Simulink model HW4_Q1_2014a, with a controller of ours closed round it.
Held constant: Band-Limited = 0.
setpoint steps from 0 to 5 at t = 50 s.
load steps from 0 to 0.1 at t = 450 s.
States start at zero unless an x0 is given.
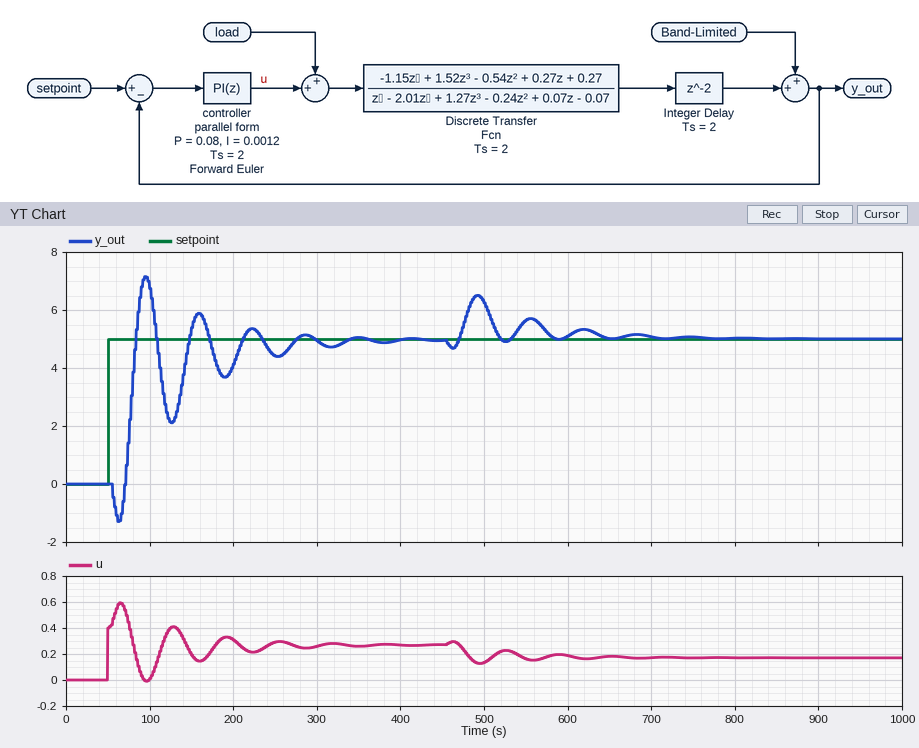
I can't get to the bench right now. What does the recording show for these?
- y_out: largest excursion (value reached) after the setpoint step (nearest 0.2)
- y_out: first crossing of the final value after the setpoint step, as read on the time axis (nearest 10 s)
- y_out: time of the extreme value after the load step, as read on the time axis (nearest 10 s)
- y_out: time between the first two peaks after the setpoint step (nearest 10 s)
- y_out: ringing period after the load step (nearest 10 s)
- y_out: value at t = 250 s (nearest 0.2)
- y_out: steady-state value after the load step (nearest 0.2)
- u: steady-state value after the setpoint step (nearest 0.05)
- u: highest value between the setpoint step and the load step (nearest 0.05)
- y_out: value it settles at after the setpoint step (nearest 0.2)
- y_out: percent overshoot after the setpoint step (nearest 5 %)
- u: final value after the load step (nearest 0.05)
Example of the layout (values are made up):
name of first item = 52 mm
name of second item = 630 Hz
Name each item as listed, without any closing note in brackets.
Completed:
y_out: largest excursion (value reached) after the setpoint step = 7.2
y_out: first crossing of the final value after the setpoint step, as read on the time axis = 80 s
y_out: time of the extreme value after the load step, as read on the time axis = 490 s
y_out: time between the first two peaks after the setpoint step = 60 s
y_out: ringing period after the load step = 60 s
y_out: value at t = 250 s = 4.4
y_out: steady-state value after the load step = 5.0
u: steady-state value after the setpoint step = 0.25
u: highest value between the setpoint step and the load step = 0.60
y_out: value it settles at after the setpoint step = 5.0
y_out: percent overshoot after the setpoint step = 45 %
u: final value after the load step = 0.15
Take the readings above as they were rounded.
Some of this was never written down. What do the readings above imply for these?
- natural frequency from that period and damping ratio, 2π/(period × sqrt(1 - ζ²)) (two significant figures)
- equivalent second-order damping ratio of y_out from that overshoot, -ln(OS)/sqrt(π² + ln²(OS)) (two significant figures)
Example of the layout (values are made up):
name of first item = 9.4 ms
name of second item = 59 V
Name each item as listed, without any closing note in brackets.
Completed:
natural frequency from that period and damping ratio, 2π/(period × sqrt(1 - ζ²)) = 0.11 rad/s
equivalent second-order damping ratio of y_out from that overshoot, -ln(OS)/sqrt(π² + ln²(OS)) = 0.25
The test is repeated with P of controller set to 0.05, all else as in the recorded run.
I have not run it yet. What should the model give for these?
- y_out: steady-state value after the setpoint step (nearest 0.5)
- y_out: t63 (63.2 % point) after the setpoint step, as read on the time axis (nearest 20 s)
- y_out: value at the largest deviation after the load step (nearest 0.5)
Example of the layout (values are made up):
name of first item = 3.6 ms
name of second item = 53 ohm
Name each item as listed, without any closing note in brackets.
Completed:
y_out: steady-state value after the setpoint step = 5.0
y_out: t63 (63.2 % point) after the setpoint step, as read on the time axis = 80 s
y_out: value at the largest deviation after the load step = 6.5
